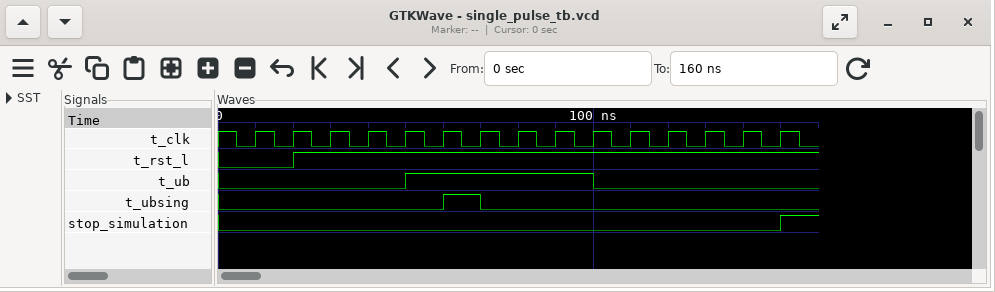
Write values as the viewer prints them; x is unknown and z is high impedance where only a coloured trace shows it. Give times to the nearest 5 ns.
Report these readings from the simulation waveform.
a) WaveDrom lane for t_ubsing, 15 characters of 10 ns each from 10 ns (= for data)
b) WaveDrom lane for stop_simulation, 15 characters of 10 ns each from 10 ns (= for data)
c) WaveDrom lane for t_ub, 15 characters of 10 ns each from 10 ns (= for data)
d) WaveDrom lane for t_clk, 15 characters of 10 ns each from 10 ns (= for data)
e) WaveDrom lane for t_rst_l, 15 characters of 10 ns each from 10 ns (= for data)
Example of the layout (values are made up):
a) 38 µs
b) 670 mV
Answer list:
a) {name: 't_ubsing', wave: '0....10........'}
b) {name: 'stop_simulation', wave: '0.............1'}
c) {name: 't_ub', wave: '0...1....0.....'}
d) {name: 't_clk', wave: 'p..............'}
e) {name: 't_rst_l', wave: '01.............'}
